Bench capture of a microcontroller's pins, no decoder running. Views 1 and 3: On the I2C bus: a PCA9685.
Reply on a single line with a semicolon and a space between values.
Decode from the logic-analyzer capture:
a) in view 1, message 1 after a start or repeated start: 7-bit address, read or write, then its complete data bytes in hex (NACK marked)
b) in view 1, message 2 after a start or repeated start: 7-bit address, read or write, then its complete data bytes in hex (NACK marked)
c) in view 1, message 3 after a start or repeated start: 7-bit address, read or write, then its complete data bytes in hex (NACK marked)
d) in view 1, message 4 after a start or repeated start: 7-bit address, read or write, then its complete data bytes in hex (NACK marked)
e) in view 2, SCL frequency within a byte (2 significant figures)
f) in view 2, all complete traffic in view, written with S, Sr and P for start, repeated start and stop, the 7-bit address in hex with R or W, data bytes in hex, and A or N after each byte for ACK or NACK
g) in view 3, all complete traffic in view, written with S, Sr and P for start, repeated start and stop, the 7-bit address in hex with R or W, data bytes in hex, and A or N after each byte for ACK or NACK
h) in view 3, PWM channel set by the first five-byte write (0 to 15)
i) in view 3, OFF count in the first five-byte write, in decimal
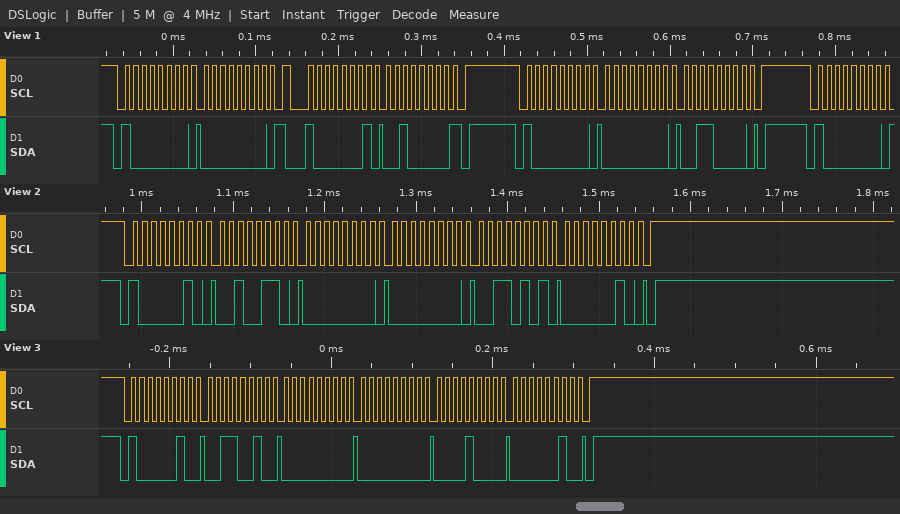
0x40 write: 00; 0x40 read: 20 NACK; 0x40 write: 00 30; 0x40 write; 100 kHz; S 41W A 26 A 00 A 00 A 35 A 02 A P; S 41W A 32 A 00 A 00 A 08 A 02 A P; 11; 520
